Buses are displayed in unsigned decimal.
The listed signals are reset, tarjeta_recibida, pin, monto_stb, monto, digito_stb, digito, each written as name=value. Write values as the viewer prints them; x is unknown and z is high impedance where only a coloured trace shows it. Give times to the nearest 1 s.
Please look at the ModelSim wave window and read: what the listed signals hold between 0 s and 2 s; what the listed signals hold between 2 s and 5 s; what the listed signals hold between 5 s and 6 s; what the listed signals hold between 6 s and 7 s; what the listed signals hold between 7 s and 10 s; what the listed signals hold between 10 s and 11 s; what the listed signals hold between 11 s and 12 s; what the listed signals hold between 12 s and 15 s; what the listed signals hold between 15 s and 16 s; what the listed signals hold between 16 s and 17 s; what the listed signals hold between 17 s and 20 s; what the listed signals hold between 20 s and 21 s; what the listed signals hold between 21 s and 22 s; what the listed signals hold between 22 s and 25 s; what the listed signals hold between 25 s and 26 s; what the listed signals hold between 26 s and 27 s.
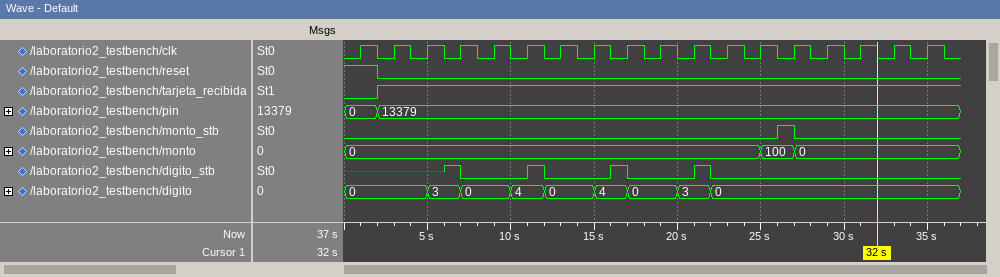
reset=1, tarjeta_recibida=0, pin=0, monto_stb=0, monto=0, digito_stb=x, digito=0
reset=0, tarjeta_recibida=1, pin=13379, monto_stb=0, monto=0, digito_stb=x, digito=0
reset=0, tarjeta_recibida=1, pin=13379, monto_stb=0, monto=0, digito_stb=x, digito=3
reset=0, tarjeta_recibida=1, pin=13379, monto_stb=0, monto=0, digito_stb=1, digito=3
reset=0, tarjeta_recibida=1, pin=13379, monto_stb=0, monto=0, digito_stb=0, digito=0
reset=0, tarjeta_recibida=1, pin=13379, monto_stb=0, monto=0, digito_stb=0, digito=4
reset=0, tarjeta_recibida=1, pin=13379, monto_stb=0, monto=0, digito_stb=1, digito=4
reset=0, tarjeta_recibida=1, pin=13379, monto_stb=0, monto=0, digito_stb=0, digito=0
reset=0, tarjeta_recibida=1, pin=13379, monto_stb=0, monto=0, digito_stb=0, digito=4
reset=0, tarjeta_recibida=1, pin=13379, monto_stb=0, monto=0, digito_stb=1, digito=4
reset=0, tarjeta_recibida=1, pin=13379, monto_stb=0, monto=0, digito_stb=0, digito=0
reset=0, tarjeta_recibida=1, pin=13379, monto_stb=0, monto=0, digito_stb=0, digito=3
reset=0, tarjeta_recibida=1, pin=13379, monto_stb=0, monto=0, digito_stb=1, digito=3
reset=0, tarjeta_recibida=1, pin=13379, monto_stb=0, monto=0, digito_stb=0, digito=0
reset=0, tarjeta_recibida=1, pin=13379, monto_stb=0, monto=100, digito_stb=0, digito=0
reset=0, tarjeta_recibida=1, pin=13379, monto_stb=1, monto=100, digito_stb=0, digito=0
